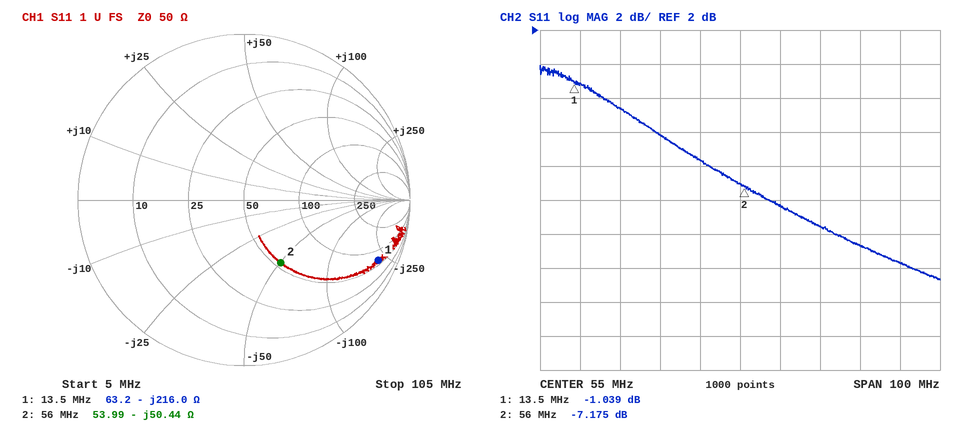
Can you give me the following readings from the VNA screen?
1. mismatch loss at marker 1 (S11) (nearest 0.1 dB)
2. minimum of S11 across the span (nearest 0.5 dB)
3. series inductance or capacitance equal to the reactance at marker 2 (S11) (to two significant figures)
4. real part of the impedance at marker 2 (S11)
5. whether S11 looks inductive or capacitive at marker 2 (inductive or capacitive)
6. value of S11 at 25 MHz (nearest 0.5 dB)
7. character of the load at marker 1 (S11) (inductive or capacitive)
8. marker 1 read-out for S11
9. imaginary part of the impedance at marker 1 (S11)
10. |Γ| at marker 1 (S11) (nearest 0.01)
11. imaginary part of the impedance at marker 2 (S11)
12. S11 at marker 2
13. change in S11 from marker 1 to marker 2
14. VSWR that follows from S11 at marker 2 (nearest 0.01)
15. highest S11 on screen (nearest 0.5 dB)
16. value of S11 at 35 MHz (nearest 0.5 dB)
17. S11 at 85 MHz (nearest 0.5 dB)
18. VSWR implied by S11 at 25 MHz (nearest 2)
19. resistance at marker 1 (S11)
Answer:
6.7 dB
-12.5 dB
56 pF
53.99 Ω
capacitive
-2.5 dB
capacitive
-1.039 dB
-216.0 Ω
0.89
-50.44 Ω
-7.175 dB
-6.136 dB
2.56
0.0 dB
-4.0 dB
-10.5 dB
6
63.2 Ω
